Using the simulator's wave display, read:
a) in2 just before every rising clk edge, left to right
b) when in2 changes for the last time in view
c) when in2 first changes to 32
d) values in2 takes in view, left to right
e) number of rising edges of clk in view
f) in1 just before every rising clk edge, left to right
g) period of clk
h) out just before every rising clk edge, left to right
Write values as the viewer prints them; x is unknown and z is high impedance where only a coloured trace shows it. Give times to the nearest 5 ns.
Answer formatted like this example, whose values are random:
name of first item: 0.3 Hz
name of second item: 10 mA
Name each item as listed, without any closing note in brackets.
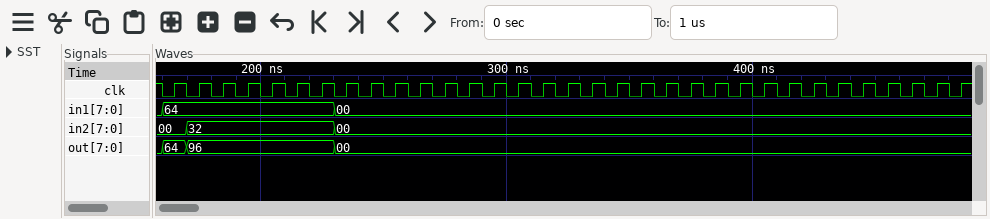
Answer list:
in2 just before every rising clk edge, left to right: 00, 32, 32, 32, 32, 32, 32, 00, 00, 00, 00, 00, 00, 00, 00, 00, 00, 00, 00, 00, 00, 00, 00, 00, 00, 00, 00, 00, 00, 00, 00, 00, 00
when in2 changes for the last time in view: 230 ns
when in2 first changes to 32: 170 ns
values in2 takes in view, left to right: 00, 32, 00
number of rising edges of clk in view: 33
in1 just before every rising clk edge, left to right: 64, 64, 64, 64, 64, 64, 64, 00, 00, 00, 00, 00, 00, 00, 00, 00, 00, 00, 00, 00, 00, 00, 00, 00, 00, 00, 00, 00, 00, 00, 00, 00, 00
period of clk: 10 ns
out just before every rising clk edge, left to right: 64, 96, 96, 96, 96, 96, 96, 00, 00, 00, 00, 00, 00, 00, 00, 00, 00, 00, 00, 00, 00, 00, 00, 00, 00, 00, 00, 00, 00, 00, 00, 00, 00
